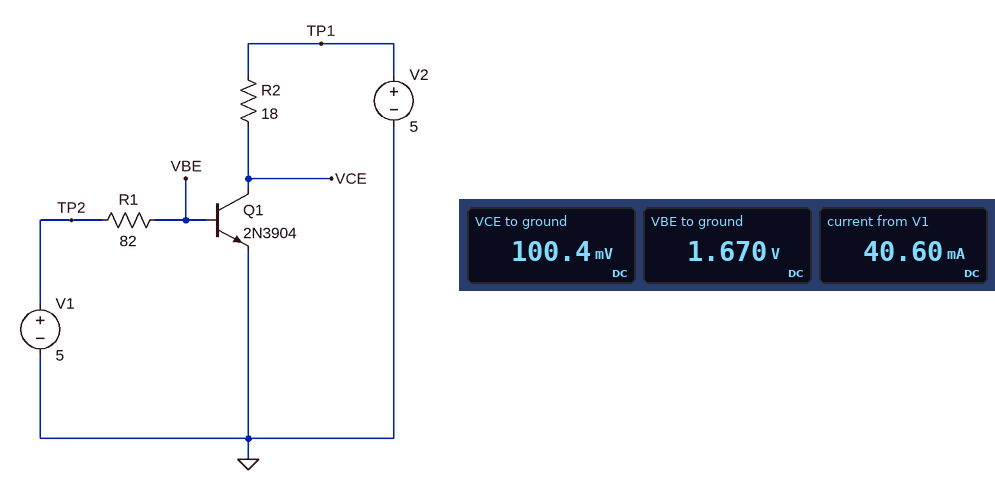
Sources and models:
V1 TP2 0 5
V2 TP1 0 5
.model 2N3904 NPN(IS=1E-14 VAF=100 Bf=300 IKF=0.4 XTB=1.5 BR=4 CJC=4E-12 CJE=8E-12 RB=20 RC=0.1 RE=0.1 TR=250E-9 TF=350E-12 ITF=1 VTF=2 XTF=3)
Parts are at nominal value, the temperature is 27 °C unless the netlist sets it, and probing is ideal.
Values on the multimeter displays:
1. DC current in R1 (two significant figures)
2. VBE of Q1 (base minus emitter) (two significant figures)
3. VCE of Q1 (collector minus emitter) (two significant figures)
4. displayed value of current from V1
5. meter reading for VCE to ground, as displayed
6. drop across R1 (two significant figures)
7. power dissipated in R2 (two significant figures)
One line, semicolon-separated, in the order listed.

41 mA; 1.7 V; 100 mV; 40.60 mA; 100.4 mV; 3.3 V; 1.3 W
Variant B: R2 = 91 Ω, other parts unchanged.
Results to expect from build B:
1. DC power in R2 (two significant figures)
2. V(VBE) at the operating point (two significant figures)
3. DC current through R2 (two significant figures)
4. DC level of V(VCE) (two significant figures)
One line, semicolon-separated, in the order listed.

270 mW; 1.6 V; 55 mA; 32 mV
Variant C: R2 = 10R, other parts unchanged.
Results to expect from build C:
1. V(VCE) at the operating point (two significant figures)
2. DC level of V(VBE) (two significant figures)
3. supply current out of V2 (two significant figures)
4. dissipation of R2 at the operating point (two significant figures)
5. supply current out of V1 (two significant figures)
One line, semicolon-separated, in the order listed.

160 mV; 1.7 V; 480 mA; 2.3 W; 40 mA
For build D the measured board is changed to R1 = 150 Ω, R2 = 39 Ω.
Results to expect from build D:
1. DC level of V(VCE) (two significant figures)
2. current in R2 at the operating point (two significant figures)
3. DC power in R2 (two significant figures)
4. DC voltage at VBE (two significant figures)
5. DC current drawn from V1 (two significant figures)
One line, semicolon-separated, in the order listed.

60 mV; 130 mA; 630 mW; 1.3 V; 25 mA
